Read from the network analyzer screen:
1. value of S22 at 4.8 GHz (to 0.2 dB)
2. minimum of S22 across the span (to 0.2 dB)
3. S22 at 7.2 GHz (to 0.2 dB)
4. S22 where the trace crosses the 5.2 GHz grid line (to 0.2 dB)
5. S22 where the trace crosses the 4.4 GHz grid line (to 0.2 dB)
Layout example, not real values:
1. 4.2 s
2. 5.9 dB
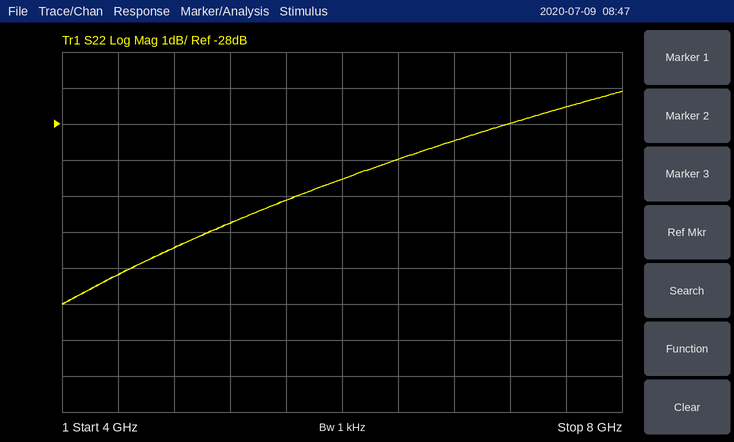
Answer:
1. -31.4 dB
2. -33.0 dB
3. -28.0 dB
4. -30.8 dB
5. -32.2 dB
